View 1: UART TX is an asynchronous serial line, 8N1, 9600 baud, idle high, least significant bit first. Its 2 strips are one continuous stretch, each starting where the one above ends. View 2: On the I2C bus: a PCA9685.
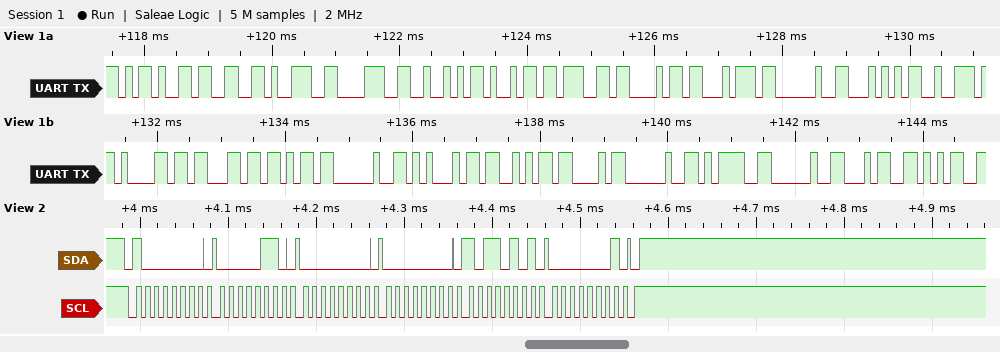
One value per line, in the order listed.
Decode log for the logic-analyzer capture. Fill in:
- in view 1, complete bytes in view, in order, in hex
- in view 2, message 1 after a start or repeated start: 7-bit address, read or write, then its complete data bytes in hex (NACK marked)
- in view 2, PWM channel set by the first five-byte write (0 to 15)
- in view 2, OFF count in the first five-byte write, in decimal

2D 33 39 38 52 69 67 68 74 20 54 72 61 63 6B 20 45 53 43 20 3D 20 34 35
0x40 write: 06 00 00 B5 01
0
437
